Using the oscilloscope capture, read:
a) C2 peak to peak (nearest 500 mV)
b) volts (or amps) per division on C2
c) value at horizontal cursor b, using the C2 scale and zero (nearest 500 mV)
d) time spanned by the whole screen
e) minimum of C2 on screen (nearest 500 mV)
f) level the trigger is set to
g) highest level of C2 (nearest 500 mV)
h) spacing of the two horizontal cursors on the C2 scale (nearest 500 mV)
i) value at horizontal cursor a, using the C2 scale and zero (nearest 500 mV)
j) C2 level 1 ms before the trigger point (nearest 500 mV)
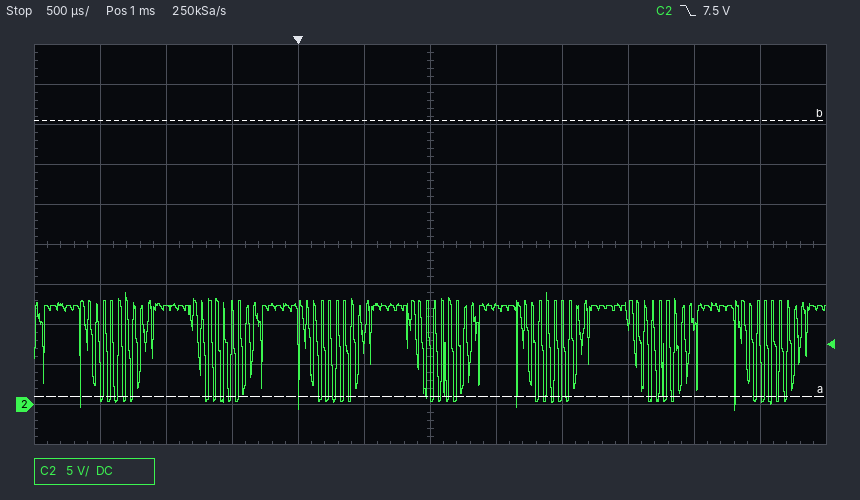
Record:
15.0 V
5 V
35.5 V
6 ms
-1.0 V
7.5 V
14.0 V
34.5 V
1.0 V
12.0 V
